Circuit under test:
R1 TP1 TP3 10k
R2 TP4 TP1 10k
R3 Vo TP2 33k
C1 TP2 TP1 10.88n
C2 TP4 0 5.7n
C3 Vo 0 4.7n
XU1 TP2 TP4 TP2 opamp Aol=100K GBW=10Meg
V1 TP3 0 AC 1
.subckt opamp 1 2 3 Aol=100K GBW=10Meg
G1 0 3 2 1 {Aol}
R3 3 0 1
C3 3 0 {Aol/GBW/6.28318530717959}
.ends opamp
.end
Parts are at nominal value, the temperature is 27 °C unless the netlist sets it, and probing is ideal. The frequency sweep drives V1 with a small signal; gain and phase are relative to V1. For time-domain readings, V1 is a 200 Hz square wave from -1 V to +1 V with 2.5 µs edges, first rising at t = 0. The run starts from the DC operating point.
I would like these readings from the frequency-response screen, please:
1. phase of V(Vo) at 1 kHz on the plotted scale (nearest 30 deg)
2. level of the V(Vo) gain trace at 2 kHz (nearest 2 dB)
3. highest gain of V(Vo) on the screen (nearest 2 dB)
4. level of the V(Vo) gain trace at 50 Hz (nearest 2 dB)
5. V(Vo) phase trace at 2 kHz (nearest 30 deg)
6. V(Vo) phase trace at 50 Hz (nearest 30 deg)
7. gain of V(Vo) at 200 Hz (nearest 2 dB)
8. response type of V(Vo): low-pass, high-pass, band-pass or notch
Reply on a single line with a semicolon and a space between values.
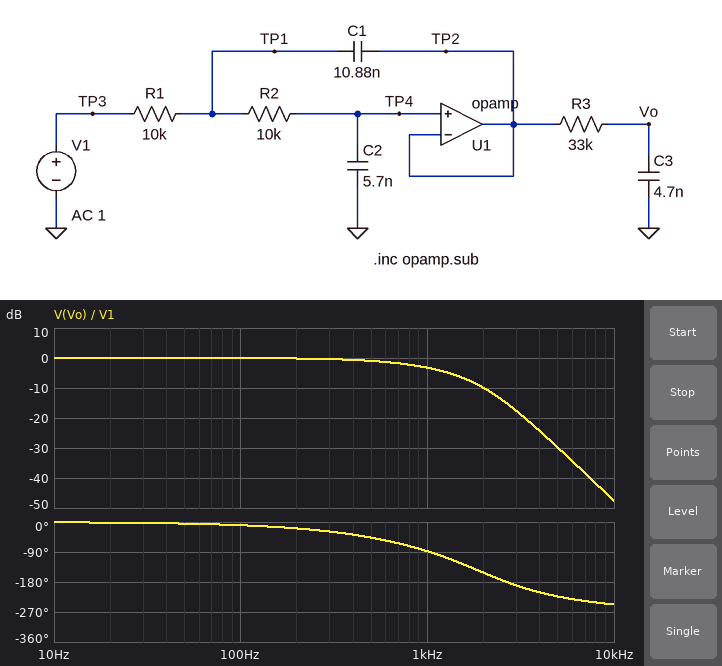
-90 deg; -10 dB; 0 dB; 0 dB; -150 deg; 0 deg; 0 dB; low-pass
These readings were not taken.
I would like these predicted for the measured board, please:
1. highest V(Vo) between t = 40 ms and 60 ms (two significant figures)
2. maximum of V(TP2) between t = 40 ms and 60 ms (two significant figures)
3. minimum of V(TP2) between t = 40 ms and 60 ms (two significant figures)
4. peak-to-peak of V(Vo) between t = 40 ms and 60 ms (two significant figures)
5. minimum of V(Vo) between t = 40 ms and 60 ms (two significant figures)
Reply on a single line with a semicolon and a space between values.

1.0 V; 1.1 V; -1.1 V; 2.0 V; -1.0 V
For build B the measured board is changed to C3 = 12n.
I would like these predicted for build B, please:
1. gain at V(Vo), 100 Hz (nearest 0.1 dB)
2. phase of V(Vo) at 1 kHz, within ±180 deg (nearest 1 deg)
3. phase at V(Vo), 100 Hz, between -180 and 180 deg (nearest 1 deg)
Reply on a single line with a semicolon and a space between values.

-0.3 dB; -112 deg; -18 deg
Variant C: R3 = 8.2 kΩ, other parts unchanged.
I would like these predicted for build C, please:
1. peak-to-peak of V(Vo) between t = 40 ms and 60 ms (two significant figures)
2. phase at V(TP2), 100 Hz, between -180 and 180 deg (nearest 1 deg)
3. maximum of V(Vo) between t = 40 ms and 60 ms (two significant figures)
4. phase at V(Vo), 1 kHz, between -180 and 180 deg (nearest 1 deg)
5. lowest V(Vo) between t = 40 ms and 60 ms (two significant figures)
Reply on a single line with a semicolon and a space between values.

2.1 V; -4 deg; 1.1 V; -57 deg; -1.1 V
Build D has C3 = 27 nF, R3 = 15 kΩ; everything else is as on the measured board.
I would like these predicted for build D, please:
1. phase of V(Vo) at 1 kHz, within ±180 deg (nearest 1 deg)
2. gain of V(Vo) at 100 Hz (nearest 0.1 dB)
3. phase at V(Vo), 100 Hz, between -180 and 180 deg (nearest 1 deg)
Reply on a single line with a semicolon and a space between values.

-112 deg; -0.3 dB; -18 deg
